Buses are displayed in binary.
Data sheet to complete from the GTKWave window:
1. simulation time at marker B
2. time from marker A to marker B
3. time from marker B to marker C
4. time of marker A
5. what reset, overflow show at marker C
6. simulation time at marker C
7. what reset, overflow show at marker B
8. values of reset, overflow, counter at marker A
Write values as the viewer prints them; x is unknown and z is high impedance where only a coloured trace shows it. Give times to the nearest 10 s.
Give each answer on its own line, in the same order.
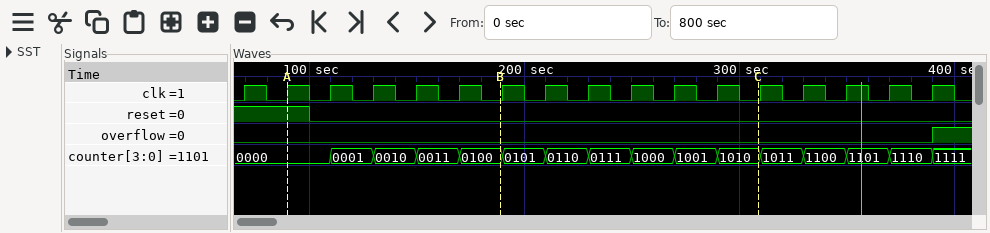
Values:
190 s
100 s
120 s
90 s
reset=0, overflow=0
310 s
reset=0, overflow=0
reset=1, overflow=0, counter=0000
